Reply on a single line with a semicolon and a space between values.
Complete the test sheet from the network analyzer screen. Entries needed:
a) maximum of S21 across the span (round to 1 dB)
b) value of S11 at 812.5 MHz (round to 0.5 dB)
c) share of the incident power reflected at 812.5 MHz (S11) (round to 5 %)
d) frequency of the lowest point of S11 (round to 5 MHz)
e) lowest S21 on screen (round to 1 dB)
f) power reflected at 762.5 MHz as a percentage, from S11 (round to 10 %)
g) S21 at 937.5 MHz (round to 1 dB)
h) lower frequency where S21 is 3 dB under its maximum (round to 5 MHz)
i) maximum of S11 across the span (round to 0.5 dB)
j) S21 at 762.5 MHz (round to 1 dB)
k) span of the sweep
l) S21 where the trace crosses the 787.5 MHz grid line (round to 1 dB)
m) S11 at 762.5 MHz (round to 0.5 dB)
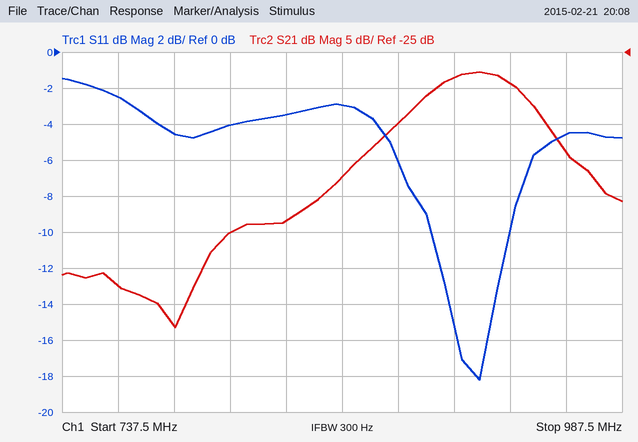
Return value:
-28 dB; -4.0 dB; 40 %; 925 MHz; -63 dB; 60 %; -29 dB; 900 MHz; -1.5 dB; -57 dB; 250 MHz; -63 dB; -2.5 dB
